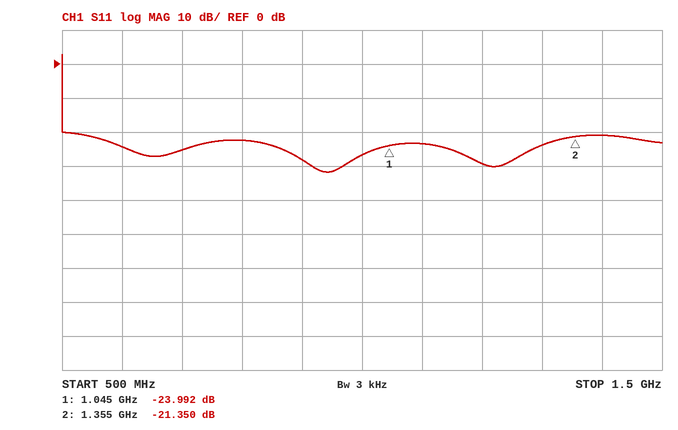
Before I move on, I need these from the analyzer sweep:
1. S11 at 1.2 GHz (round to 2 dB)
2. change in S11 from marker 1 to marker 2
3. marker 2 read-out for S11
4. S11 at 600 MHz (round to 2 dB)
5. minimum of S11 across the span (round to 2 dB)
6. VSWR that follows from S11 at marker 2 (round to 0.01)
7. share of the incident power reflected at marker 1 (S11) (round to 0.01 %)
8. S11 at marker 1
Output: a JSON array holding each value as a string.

["-30 dB", "2.642 dB", "-21.350 dB", "-24 dB", "-32 dB", "1.19", "0.40 %", "-23.992 dB"]
